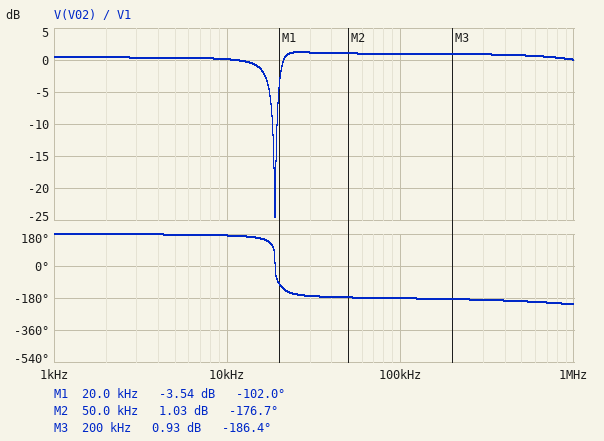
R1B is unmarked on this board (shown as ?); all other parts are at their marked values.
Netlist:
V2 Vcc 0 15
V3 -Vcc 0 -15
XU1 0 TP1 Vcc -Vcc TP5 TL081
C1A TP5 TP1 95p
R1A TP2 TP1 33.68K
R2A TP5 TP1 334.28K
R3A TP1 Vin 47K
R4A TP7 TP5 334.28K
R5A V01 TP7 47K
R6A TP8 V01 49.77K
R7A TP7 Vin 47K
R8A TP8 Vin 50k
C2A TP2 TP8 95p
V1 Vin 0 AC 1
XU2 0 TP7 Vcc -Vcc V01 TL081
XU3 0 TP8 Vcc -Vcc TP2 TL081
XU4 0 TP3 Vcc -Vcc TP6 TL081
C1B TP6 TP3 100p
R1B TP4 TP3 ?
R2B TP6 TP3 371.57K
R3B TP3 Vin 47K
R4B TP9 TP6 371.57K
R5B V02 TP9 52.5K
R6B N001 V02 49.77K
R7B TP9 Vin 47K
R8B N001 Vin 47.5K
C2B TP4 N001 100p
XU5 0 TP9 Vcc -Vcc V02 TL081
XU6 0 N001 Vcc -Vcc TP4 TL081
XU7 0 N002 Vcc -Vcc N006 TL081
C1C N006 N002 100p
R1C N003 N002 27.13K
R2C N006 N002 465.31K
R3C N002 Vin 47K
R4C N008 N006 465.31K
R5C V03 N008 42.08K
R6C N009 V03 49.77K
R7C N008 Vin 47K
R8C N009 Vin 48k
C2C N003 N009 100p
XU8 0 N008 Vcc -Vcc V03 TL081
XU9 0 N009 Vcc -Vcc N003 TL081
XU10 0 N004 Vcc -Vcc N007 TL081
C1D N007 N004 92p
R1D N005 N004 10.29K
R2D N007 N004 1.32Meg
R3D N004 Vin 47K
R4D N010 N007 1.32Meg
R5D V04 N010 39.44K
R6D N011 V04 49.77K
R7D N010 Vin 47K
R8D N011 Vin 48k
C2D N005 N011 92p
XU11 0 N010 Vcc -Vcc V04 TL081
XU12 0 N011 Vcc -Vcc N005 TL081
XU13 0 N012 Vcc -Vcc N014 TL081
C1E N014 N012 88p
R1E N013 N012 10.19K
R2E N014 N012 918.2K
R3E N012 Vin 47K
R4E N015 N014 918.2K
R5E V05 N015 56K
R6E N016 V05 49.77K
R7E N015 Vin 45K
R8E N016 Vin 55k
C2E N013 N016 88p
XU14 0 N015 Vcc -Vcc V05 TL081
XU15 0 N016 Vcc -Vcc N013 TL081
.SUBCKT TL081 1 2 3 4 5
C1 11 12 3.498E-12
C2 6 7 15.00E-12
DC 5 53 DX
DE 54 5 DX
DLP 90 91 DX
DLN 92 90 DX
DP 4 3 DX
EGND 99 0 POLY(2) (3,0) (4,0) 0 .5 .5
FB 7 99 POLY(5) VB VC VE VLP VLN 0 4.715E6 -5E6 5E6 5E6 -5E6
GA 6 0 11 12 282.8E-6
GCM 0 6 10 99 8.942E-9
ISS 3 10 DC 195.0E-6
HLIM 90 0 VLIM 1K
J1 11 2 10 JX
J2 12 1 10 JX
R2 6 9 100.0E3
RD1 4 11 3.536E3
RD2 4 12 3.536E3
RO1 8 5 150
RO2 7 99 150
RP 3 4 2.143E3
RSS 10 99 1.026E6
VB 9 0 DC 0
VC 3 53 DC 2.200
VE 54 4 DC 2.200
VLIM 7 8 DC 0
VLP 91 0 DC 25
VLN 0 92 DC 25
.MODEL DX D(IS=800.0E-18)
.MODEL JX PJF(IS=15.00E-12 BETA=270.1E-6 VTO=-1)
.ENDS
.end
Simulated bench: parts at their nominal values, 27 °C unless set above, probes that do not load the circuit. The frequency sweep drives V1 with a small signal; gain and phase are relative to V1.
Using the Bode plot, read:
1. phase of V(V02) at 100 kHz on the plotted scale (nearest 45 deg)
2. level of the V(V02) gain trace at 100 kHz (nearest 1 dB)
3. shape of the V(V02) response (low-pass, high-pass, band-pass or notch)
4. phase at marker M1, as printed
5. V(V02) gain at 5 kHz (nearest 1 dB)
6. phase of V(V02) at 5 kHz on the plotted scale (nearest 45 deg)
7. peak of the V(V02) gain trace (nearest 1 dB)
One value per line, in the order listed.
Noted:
-180 deg
1 dB
notch
-102.0 deg
0 dB
180 deg
1 dB
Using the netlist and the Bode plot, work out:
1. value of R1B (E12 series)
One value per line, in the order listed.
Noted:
18 kΩ
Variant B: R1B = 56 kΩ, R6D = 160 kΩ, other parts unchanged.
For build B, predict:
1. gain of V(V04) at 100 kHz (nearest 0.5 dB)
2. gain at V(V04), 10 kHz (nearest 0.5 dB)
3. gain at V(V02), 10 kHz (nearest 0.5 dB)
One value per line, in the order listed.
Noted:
-1.5 dB
4.5 dB
-8.5 dB
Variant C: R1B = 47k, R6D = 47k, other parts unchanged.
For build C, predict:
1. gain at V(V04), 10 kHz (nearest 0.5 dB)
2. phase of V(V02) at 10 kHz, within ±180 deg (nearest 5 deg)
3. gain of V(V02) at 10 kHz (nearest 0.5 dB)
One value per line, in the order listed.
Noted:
1.5 dB
140 deg
-3.5 dB
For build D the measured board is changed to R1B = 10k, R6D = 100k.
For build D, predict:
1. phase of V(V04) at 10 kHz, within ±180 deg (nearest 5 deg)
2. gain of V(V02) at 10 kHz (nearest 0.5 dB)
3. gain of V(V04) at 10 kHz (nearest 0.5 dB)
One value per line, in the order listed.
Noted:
30 deg
0.5 dB
11.5 dB
